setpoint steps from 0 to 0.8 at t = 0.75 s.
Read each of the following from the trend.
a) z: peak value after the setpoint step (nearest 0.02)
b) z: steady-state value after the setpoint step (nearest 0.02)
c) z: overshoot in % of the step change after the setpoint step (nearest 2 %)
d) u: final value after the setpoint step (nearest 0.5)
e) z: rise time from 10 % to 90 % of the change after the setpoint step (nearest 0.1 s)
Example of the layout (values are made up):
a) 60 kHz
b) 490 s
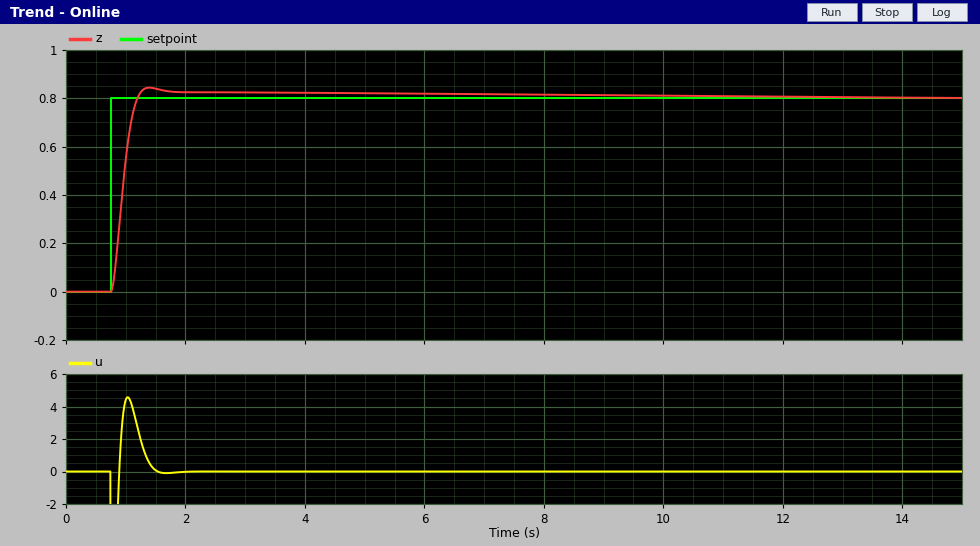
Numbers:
a) 0.84
b) 0.80
c) 6 %
d) 0.0
e) 0.3 s
